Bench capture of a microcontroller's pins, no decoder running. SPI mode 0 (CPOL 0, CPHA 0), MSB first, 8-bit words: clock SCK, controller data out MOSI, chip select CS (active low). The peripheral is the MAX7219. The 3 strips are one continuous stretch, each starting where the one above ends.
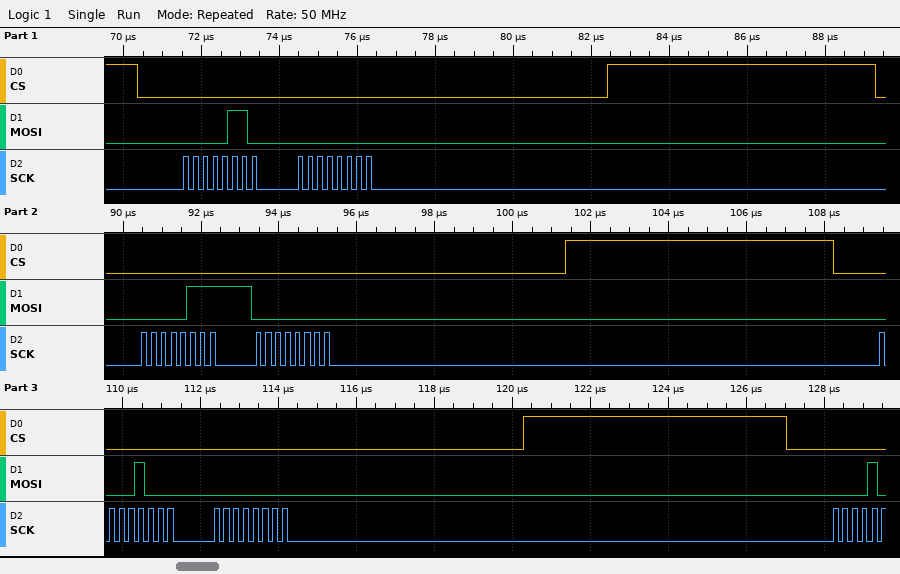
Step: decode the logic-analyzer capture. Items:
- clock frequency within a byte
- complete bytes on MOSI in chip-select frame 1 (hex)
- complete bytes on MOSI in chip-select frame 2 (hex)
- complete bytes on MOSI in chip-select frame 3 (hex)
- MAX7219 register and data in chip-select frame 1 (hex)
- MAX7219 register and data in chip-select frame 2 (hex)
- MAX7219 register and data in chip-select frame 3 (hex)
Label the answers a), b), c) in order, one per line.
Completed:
a) 4 MHz
b) 0x06 0x00
c) 0x07 0x00
d) 0x08 0x00
e) register 0x6, data 0x00
f) register 0x7, data 0x00
g) register 0x8, data 0x00
